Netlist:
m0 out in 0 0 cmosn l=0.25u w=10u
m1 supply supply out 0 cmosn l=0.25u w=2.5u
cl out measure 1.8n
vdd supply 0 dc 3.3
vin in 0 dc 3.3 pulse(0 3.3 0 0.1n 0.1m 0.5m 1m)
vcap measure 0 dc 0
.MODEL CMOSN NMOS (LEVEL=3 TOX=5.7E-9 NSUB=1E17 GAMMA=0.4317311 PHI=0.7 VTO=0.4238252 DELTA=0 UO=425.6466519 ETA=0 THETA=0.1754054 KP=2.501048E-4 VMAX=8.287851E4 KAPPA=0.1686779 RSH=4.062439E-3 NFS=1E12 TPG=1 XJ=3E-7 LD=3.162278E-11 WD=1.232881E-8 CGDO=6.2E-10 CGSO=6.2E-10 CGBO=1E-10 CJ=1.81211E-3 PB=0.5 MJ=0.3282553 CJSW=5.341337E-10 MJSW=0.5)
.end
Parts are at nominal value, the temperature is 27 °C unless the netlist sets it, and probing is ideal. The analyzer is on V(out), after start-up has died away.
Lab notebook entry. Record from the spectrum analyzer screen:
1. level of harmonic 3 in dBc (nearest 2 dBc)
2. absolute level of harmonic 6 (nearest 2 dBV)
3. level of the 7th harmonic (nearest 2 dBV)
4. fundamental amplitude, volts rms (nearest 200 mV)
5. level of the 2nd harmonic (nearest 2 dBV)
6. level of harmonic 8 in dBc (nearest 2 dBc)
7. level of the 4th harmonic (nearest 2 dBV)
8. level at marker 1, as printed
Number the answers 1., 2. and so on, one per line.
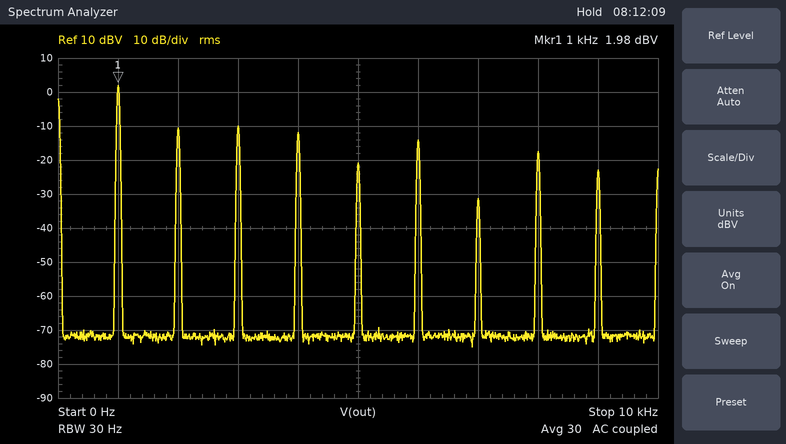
1. -12 dBc
2. -14 dBV
3. -32 dBV
4. 1.2 V
5. -10 dBV
6. -20 dBc
7. -12 dBV
8. 1.98 dBV
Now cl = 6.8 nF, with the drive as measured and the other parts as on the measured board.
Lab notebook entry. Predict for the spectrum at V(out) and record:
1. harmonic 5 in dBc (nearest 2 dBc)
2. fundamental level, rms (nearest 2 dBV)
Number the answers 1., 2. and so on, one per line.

1. -24 dBc
2. 2 dBV
